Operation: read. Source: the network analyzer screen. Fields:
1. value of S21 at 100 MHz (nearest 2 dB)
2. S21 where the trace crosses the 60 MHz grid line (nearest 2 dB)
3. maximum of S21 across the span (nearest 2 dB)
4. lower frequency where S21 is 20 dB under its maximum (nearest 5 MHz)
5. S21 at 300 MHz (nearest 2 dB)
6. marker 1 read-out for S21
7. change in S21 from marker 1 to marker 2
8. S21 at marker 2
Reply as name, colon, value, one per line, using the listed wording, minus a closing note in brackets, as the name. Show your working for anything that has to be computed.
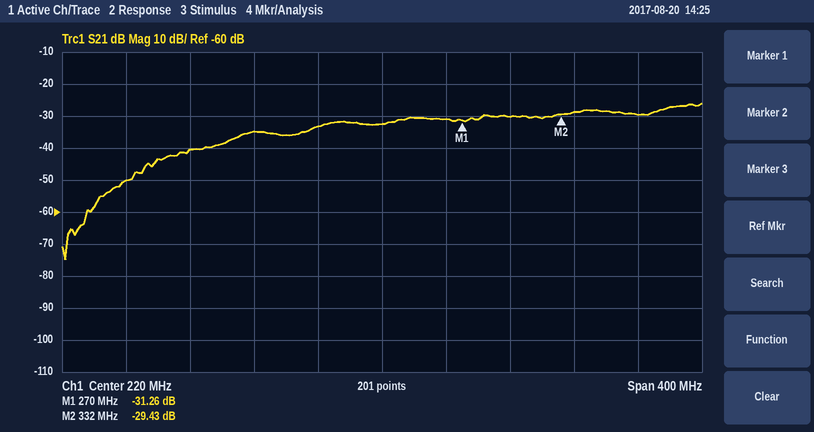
value of S21 at 100 MHz: -40 dB
S21 where the trace crosses the 60 MHz grid line: -50 dB
maximum of S21 across the span: -26 dB
lower frequency where S21 is 20 dB under its maximum: 70 MHz
S21 at 300 MHz: -30 dB
marker 1 read-out for S21: -31.26 dB
change in S21 from marker 1 to marker 2: -29.43 − (-31.26) = 1.83 dB
S21 at marker 2: -29.43 dB
